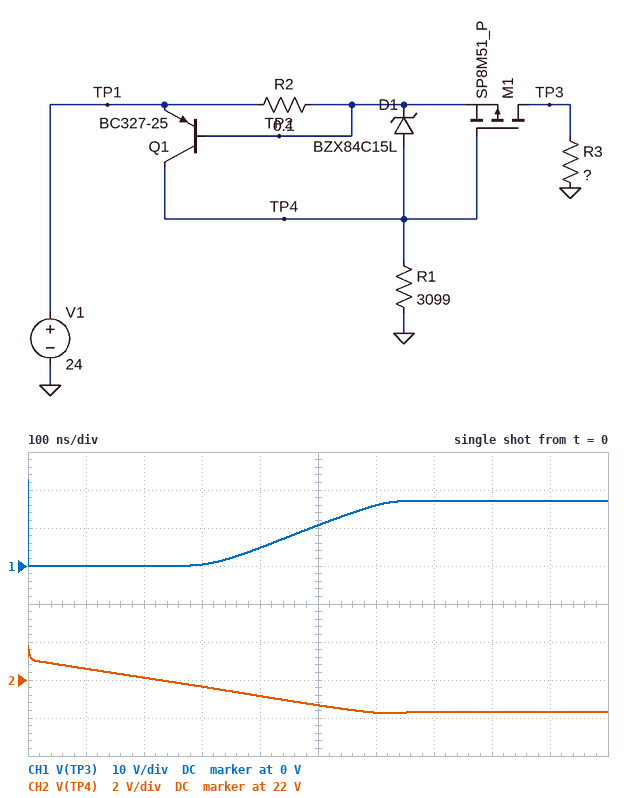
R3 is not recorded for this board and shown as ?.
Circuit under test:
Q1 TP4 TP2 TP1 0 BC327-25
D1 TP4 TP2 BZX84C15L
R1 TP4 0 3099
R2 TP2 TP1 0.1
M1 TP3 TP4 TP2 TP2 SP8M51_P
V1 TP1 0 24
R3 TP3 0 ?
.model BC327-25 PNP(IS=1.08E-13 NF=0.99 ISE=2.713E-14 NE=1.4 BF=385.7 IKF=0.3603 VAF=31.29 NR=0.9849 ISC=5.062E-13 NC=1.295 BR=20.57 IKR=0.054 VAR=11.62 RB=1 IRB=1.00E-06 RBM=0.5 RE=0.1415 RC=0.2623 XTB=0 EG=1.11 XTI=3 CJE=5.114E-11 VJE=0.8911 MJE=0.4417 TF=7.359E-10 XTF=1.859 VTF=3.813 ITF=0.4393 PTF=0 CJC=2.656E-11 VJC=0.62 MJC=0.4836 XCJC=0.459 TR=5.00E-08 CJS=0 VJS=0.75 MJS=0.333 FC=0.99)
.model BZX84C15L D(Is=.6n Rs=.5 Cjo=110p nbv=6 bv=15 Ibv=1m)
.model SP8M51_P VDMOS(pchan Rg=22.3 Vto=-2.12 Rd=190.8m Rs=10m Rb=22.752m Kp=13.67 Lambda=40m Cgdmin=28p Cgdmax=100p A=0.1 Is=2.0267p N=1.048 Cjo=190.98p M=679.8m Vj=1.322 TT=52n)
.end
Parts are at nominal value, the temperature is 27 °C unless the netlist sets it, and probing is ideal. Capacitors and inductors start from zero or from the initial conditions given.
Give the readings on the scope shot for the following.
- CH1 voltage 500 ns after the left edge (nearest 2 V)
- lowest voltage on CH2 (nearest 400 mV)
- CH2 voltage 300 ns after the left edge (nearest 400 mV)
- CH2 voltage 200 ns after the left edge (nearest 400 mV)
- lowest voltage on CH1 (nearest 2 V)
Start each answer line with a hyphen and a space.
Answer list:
- 10 V
- 20.4 V
- 21.6 V
- 22.0 V
- 0 V
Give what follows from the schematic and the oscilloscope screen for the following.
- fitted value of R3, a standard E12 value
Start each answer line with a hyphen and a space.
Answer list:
- 2.7 Ω
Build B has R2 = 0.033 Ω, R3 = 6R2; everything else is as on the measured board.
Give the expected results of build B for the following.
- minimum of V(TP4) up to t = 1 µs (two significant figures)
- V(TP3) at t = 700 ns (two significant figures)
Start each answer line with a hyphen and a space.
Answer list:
- 19 V
- 23 V
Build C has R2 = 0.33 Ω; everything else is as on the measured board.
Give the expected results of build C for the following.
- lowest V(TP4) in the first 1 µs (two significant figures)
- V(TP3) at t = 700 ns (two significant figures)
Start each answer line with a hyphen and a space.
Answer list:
- 21 V
- 5.2 V
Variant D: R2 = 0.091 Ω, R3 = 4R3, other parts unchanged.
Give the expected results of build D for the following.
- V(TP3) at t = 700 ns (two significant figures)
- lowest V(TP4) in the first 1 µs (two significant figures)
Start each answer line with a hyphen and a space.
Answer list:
- 22 V
- 19 V
